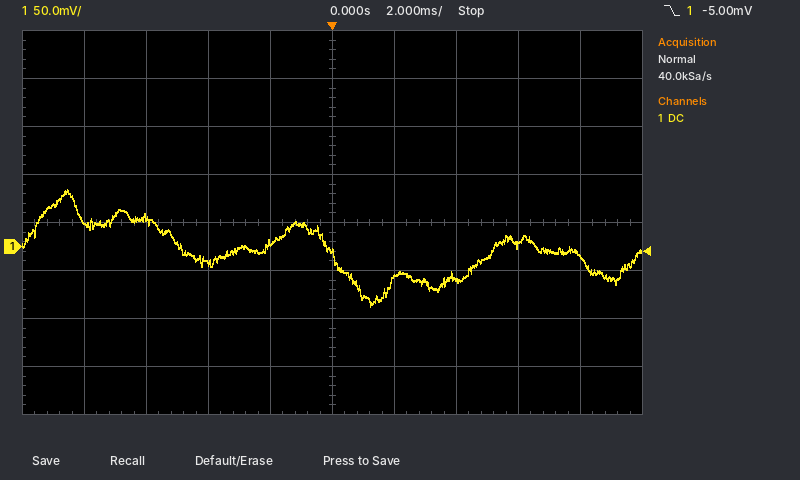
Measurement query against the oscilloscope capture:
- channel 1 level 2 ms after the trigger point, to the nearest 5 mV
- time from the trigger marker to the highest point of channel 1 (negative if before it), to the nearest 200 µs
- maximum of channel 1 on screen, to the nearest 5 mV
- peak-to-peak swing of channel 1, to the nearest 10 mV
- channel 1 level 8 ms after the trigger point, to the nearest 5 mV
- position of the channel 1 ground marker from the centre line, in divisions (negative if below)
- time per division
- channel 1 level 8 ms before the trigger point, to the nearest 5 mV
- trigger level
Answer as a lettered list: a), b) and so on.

a) -35 mV
b) -8.6 ms
c) 60 mV
d) 120 mV
e) -10 mV
f) -0.5 div
g) 2 ms
h) 25 mV
i) -5.00 mV
